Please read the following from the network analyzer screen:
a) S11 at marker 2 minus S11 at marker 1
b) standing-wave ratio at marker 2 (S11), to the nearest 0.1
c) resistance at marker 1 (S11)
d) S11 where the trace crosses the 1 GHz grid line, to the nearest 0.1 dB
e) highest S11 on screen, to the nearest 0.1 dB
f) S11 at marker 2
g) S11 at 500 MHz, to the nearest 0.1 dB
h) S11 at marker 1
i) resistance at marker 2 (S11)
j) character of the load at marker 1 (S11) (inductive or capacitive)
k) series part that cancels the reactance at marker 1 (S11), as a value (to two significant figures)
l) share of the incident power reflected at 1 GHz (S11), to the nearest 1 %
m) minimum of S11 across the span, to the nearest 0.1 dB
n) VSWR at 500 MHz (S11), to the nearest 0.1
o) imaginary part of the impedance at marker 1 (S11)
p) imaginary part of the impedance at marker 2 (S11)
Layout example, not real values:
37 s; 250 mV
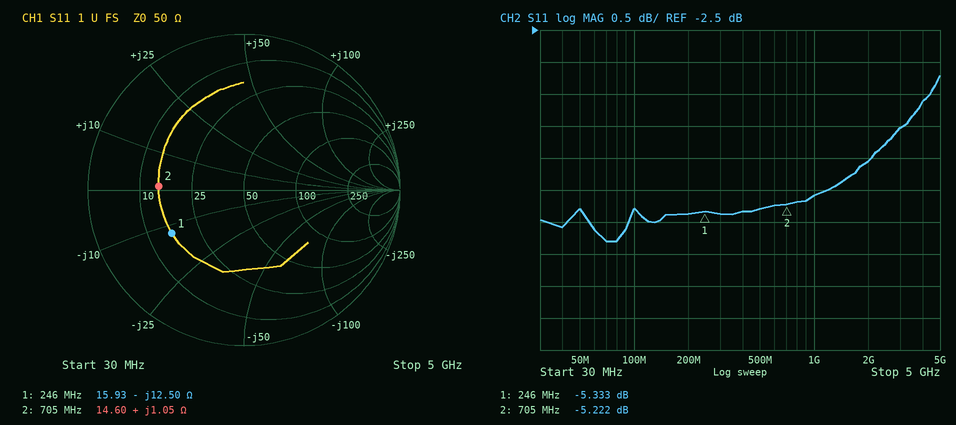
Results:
0.111 dB; 3.4; 15.93 Ω; -5.1 dB; -3.2 dB; -5.222 dB; -5.3 dB; -5.333 dB; 14.60 Ω; capacitive; 8.1 nH; 31 %; -5.8 dB; 3.4; -12.50 Ω; +1.05 Ω
